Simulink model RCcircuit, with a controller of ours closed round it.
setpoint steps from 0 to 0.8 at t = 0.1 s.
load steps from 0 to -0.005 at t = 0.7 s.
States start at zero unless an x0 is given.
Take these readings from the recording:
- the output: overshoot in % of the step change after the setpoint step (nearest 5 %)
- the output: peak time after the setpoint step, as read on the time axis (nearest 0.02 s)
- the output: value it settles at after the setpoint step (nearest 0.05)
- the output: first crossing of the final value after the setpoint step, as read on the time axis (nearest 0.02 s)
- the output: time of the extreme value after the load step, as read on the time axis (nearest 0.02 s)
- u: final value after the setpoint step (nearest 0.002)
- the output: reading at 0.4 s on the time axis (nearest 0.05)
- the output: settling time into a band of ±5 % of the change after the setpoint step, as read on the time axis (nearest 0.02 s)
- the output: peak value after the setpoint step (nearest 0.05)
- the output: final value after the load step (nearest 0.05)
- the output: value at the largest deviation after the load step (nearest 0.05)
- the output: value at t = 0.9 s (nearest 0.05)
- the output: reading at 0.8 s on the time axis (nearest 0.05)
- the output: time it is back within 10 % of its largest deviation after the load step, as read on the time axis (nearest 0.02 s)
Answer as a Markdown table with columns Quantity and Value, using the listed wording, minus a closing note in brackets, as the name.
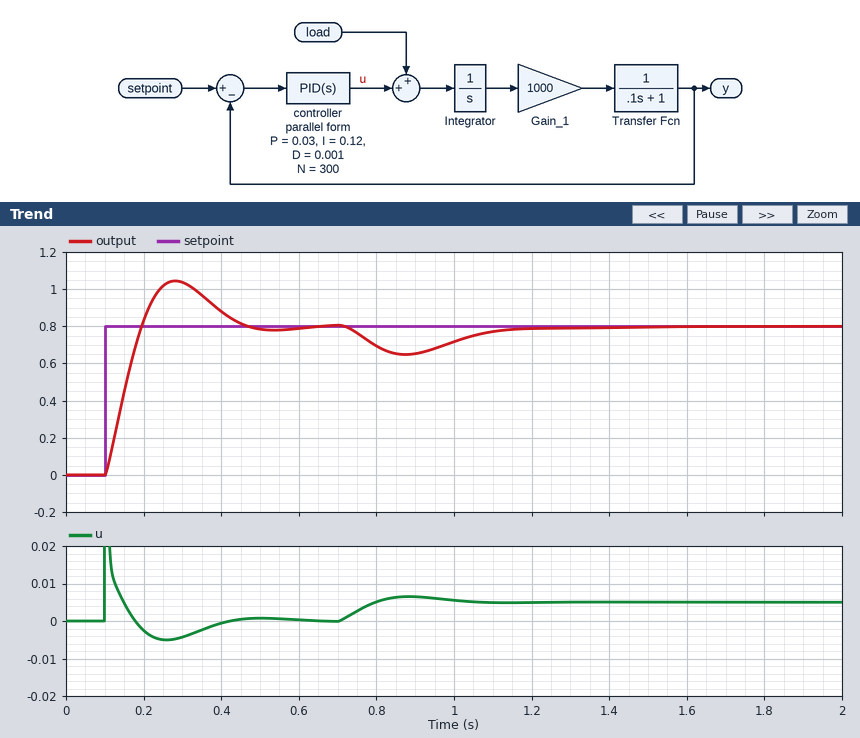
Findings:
| Quantity | Value |
|---|---|
| the output: overshoot in % of the step change after the setpoint step | 30 % |
| the output: peak time after the setpoint step, as read on the time axis | 0.28 s |
| the output: value it settles at after the setpoint step | 0.80 |
| the output: first crossing of the final value after the setpoint step, as read on the time axis | 0.20 s |
| the output: time of the extreme value after the load step, as read on the time axis | 0.88 s |
| u: final value after the setpoint step | 0.000 |
| the output: reading at 0.4 s on the time axis | 0.90 |
| the output: settling time into a band of ±5 % of the change after the setpoint step, as read on the time axis | 0.42 s |
| the output: peak value after the setpoint step | 1.05 |
| the output: final value after the load step | 0.80 |
| the output: value at the largest deviation after the load step | 0.65 |
| the output: value at t = 0.9 s | 0.65 |
| the output: reading at 0.8 s on the time axis | 0.70 |
| the output: time it is back within 10 % of its largest deviation after the load step, as read on the time axis | 1.16 s |
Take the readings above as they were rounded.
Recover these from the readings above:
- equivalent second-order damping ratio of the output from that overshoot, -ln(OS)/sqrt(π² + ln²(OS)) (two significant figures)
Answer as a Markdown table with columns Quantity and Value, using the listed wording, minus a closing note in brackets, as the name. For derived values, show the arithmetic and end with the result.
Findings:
| Quantity | Value |
|---|---|
| equivalent second-order damping ratio of the output from that overshoot, -ln(OS)/sqrt(π² + ln²(OS)) | ln(0.3) = -1.204; 1.204 / sqrt(9.870 + 1.450) = 0.36 |
